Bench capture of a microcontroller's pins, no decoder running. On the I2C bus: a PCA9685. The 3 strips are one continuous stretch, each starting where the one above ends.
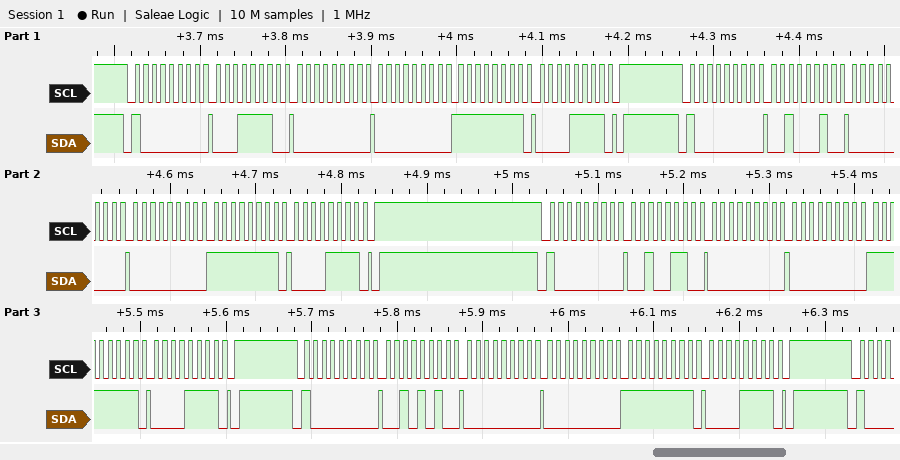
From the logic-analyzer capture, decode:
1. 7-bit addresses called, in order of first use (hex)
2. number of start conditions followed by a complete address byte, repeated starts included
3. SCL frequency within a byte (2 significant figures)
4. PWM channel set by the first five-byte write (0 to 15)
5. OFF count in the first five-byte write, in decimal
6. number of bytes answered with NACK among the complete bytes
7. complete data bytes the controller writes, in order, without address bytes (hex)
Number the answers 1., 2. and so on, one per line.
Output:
1. 0x40
2. 4
3. 100 kHz
4. 6
5. 4095
6. 0
7. 1E 00 00 FF 0F 22 00 00 FF 0F 26 00 00 FF 0F 2A 00 00 FF 0F
